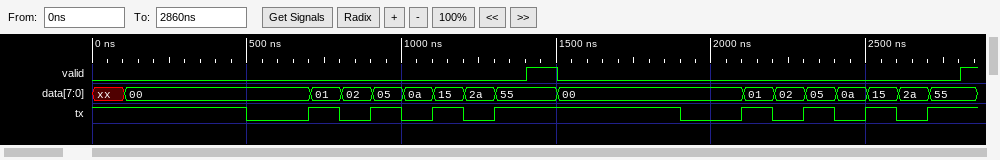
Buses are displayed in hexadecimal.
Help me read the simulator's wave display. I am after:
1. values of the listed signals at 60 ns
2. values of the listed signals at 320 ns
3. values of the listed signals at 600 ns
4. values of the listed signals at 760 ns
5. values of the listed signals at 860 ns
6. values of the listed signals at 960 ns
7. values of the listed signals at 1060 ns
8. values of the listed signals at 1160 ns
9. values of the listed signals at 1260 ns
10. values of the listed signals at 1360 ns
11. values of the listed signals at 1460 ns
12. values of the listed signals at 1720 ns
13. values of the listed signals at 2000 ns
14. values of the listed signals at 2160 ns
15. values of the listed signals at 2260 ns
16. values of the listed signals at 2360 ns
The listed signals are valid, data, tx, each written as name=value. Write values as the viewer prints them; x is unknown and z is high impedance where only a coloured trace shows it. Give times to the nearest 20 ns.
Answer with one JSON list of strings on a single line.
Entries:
["valid=0, data=xx, tx=1", "valid=0, data=00, tx=1", "valid=0, data=00, tx=0", "valid=0, data=01, tx=1", "valid=0, data=02, tx=0", "valid=0, data=05, tx=1", "valid=0, data=0a, tx=0", "valid=0, data=15, tx=1", "valid=0, data=2a, tx=0", "valid=0, data=55, tx=1", "valid=1, data=55, tx=1", "valid=0, data=00, tx=1", "valid=0, data=00, tx=0", "valid=0, data=01, tx=1", "valid=0, data=02, tx=0", "valid=0, data=05, tx=1"]
